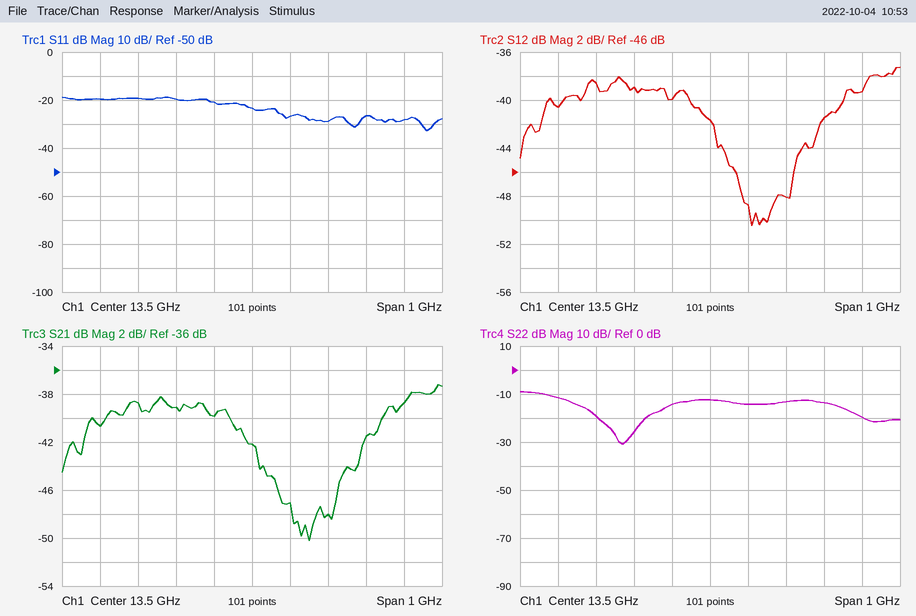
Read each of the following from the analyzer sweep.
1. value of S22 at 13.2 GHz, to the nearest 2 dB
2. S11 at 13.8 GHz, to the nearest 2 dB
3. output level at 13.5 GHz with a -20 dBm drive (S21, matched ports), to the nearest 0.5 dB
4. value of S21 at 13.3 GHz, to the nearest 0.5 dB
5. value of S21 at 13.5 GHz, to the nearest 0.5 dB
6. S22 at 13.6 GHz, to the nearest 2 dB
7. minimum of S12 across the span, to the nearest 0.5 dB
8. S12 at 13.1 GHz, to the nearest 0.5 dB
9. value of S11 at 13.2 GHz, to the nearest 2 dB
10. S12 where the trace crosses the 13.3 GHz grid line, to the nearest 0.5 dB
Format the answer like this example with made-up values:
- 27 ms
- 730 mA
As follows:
- -20 dB
- -26 dB
- -62.0 dBm
- -39.0 dB
- -42.0 dB
- -14 dB
- -50.5 dB
- -40.5 dB
- -20 dB
- -39.0 dB
